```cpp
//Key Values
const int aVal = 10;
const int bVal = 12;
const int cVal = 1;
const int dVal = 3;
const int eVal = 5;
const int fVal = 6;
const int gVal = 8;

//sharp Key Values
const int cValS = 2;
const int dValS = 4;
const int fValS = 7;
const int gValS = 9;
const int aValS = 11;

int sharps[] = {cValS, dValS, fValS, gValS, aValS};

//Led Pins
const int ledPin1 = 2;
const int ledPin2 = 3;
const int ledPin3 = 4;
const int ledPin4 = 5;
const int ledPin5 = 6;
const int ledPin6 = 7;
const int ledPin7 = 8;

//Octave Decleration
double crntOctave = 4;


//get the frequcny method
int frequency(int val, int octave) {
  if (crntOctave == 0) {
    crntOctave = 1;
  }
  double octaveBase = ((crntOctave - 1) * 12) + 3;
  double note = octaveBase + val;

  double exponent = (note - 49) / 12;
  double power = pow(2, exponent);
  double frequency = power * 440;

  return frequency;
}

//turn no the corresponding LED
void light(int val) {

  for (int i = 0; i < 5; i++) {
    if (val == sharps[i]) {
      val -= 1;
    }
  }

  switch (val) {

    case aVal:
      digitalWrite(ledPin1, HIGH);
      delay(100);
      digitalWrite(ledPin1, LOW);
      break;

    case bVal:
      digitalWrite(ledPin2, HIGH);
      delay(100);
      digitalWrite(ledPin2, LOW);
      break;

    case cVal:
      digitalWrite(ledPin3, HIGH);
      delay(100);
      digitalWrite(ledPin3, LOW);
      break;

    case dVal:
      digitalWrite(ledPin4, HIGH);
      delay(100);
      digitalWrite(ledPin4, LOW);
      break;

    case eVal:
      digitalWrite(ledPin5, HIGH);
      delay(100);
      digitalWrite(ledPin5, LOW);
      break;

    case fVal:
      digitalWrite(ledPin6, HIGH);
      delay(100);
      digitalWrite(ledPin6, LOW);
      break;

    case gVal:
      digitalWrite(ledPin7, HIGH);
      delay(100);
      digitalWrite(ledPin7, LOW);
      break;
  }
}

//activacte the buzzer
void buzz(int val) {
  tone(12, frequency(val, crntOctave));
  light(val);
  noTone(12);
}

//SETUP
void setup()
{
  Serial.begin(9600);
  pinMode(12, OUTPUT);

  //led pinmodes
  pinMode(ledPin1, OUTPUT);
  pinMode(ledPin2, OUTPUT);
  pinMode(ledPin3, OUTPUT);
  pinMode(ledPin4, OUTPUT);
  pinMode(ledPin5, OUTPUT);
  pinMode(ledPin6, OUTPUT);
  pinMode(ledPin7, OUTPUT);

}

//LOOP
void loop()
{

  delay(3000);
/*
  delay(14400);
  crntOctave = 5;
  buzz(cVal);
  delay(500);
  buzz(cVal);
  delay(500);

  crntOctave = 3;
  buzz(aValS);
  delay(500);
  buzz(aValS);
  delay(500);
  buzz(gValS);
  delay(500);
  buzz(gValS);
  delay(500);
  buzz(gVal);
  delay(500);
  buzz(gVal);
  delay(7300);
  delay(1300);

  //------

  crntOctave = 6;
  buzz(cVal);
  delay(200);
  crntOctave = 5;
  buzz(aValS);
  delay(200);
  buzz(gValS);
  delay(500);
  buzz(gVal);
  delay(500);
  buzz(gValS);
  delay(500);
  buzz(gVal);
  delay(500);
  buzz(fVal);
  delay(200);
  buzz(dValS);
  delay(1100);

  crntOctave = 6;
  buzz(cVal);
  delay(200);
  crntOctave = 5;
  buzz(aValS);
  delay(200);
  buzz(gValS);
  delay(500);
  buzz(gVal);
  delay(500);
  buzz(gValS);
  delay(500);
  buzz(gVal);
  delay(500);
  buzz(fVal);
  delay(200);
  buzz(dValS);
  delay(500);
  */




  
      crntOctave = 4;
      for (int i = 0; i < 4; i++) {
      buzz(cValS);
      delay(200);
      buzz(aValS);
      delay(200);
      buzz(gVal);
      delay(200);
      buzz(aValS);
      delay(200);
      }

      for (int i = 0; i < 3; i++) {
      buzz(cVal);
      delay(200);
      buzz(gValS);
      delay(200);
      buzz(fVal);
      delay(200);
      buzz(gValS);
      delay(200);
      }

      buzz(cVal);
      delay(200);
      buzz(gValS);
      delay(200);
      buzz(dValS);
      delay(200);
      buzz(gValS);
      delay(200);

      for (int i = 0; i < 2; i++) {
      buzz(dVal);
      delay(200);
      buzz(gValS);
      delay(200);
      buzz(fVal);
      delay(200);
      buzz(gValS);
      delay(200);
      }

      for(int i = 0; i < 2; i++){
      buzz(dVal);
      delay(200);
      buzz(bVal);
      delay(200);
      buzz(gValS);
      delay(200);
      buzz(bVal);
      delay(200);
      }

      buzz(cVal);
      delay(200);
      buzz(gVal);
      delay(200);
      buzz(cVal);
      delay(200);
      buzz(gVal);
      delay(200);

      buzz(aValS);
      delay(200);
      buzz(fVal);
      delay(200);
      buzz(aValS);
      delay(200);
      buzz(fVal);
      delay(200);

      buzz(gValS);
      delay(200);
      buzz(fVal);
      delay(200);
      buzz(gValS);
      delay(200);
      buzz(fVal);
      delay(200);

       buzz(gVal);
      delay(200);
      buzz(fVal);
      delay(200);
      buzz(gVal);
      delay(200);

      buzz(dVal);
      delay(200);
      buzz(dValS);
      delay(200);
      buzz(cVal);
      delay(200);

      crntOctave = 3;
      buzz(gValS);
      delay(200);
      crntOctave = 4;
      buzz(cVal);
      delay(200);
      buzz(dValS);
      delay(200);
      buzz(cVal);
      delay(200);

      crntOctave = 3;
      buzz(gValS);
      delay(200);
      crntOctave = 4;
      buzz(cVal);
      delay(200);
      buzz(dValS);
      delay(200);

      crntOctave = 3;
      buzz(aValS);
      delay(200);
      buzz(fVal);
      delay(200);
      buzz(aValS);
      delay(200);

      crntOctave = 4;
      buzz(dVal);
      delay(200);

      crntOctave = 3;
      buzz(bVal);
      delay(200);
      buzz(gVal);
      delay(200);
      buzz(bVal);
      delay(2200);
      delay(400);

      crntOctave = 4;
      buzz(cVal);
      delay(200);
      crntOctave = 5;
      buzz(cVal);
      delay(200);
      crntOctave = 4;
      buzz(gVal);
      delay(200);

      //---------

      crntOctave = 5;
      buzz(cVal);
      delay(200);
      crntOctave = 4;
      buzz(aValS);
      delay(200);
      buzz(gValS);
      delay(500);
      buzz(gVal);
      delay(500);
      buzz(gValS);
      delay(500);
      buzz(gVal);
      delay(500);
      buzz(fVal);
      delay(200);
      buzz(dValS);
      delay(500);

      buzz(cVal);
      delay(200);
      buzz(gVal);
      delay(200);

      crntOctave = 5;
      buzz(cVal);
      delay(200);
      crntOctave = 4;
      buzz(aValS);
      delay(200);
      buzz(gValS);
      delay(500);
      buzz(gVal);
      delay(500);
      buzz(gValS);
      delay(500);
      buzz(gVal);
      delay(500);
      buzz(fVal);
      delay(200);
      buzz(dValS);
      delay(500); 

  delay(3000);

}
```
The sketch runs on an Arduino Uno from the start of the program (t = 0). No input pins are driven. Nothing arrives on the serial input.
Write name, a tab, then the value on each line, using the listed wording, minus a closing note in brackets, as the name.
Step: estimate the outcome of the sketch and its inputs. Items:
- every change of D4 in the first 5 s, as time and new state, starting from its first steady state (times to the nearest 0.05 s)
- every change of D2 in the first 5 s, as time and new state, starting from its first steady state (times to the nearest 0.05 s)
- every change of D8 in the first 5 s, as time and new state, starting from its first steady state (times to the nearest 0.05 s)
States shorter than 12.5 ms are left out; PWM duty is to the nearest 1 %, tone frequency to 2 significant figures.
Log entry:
every change of D4 in the first 5 s, as time and new state, starting from its first steady state	0 s low; 3 s high; 3.1 s low; 4.2 s high; 4.3 s low
every change of D2 in the first 5 s, as time and new state, starting from its first steady state	0 s low; 3.3 s high; 3.4 s low; 3.9 s high; 4 s low; 4.5 s high; 4.6 s low
every change of D8 in the first 5 s, as time and new state, starting from its first steady state	0 s low; 3.6 s high; 3.7 s low; 4.8 s high; 4.9 s low
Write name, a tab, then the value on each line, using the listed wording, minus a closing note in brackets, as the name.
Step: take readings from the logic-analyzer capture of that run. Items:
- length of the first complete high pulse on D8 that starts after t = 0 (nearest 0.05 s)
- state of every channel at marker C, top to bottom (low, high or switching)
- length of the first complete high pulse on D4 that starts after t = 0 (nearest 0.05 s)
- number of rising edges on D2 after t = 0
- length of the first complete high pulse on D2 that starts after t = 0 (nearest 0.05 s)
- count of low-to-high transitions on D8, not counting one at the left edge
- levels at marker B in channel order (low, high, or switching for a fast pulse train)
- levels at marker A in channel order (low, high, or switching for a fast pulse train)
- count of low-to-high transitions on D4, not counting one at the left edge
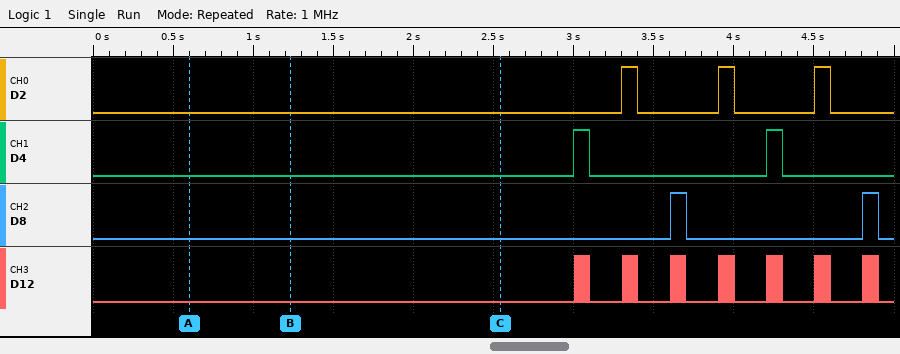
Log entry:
length of the first complete high pulse on D8 that starts after t = 0	0.10 s
state of every channel at marker C, top to bottom	D2 low, D4 low, D8 low, D12 low
length of the first complete high pulse on D4 that starts after t = 0	0.10 s
number of rising edges on D2 after t = 0	3
length of the first complete high pulse on D2 that starts after t = 0	0.10 s
count of low-to-high transitions on D8, not counting one at the left edge	2
levels at marker B in channel order	D2 low, D4 low, D8 low, D12 low
levels at marker A in channel order	D2 low, D4 low, D8 low, D12 low
count of low-to-high transitions on D4, not counting one at the left edge	2
